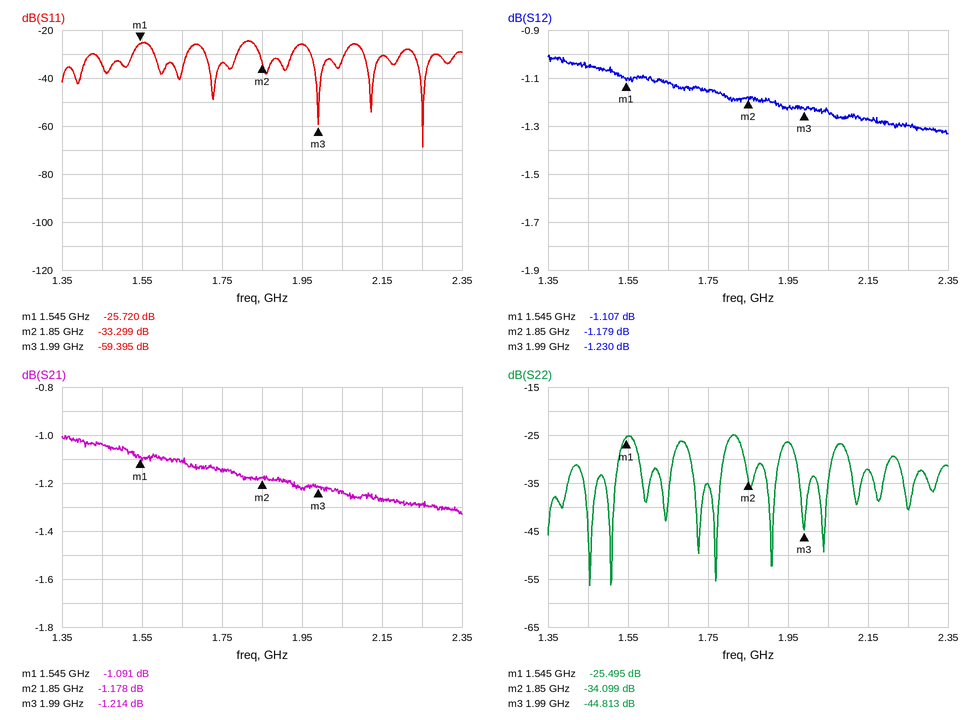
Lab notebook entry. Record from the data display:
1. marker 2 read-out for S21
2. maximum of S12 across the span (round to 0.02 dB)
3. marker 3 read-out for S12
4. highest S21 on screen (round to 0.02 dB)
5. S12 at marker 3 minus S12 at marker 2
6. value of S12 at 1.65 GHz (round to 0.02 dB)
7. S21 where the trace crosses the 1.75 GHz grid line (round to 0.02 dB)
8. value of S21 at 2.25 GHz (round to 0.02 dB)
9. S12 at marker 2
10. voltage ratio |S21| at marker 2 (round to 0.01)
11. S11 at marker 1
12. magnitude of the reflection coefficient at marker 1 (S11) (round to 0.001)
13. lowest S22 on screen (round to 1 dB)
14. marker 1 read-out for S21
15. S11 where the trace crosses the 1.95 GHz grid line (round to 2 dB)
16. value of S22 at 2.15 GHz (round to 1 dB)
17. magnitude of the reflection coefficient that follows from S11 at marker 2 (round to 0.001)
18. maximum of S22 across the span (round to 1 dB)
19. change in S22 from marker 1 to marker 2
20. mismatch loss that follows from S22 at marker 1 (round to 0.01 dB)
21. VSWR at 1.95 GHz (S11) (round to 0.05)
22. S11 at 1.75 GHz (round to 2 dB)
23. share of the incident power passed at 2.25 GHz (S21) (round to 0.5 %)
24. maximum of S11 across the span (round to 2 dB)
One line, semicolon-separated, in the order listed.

-1.178 dB; -1.00 dB; -1.230 dB; -1.00 dB; -0.051 dB; -1.12 dB; -1.14 dB; -1.28 dB; -1.179 dB; 0.87; -25.720 dB; 0.052; -56 dB; -1.091 dB; -26 dB; -32 dB; 0.022; -25 dB; -8.604 dB; 0.01 dB; 1.10; -34 dB; 74.5 %; -24 dB
